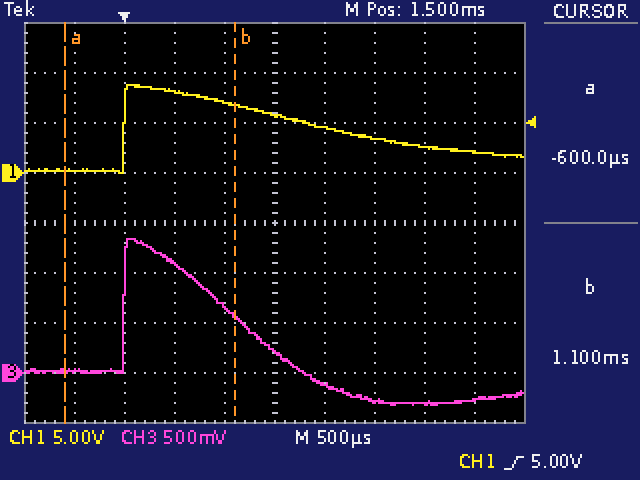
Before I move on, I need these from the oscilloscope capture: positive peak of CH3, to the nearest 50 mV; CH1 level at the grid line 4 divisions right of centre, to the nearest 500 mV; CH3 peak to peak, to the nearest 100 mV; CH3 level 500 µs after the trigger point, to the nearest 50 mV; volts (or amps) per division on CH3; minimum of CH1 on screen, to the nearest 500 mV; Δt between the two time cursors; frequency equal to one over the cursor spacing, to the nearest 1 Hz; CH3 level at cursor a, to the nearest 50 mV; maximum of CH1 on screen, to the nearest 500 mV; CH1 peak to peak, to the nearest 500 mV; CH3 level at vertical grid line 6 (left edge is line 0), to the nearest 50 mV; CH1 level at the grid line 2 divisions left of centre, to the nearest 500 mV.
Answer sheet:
1.35 V
2.0 V
1.70 V
1.10 V
500 mV
0.0 V
1.70 ms
588 Hz
0 mV
9.0 V
9.0 V
-100 mV
8.0 V
